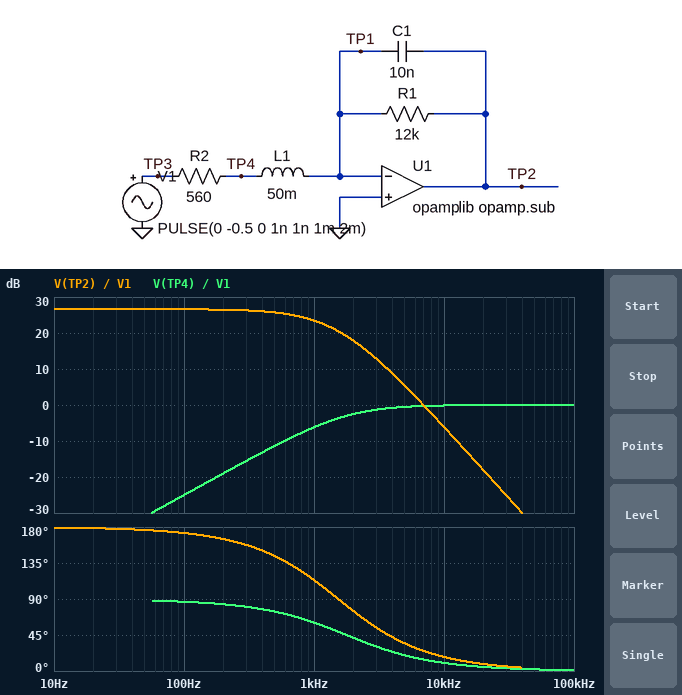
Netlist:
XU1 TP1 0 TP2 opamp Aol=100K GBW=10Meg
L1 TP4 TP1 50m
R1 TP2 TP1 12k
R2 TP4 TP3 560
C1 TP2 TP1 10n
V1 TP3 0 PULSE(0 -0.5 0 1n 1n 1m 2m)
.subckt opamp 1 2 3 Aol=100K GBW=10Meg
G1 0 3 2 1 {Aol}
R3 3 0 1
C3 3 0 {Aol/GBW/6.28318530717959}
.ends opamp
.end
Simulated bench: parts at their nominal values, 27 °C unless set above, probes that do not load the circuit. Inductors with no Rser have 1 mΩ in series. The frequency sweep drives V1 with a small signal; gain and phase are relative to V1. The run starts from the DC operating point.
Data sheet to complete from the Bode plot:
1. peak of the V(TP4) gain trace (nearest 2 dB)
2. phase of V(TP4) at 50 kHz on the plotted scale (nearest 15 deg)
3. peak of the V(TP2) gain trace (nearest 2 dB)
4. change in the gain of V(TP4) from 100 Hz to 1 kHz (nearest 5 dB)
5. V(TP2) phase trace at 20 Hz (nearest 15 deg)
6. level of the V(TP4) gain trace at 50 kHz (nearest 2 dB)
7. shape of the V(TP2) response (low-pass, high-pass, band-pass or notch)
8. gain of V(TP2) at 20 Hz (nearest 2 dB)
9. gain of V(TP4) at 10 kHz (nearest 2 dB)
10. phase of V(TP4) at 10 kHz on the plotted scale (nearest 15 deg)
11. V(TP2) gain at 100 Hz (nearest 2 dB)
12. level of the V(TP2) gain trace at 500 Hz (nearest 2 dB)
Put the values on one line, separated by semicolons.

0 dB; 0 deg; 26 dB; 20 dB; 180 deg; 0 dB; low-pass; 26 dB; 0 dB; 15 deg; 26 dB; 26 dB
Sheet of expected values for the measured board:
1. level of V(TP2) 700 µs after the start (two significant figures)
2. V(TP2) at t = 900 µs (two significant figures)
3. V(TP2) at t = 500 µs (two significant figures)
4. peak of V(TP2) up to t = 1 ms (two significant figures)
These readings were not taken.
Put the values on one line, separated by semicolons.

11 V; 11 V; 10 V; 11 V
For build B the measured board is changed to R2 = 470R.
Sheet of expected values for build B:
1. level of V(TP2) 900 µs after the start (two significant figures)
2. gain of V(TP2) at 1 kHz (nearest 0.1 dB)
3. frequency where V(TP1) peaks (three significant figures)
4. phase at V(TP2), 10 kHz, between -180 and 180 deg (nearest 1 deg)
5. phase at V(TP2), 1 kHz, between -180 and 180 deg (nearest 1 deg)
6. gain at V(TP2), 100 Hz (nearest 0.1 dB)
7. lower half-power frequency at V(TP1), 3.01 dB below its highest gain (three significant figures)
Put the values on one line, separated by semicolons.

13 V; 24.6 dB; 1.40 kHz; 16 deg; 109 deg; 28.1 dB; 572 Hz
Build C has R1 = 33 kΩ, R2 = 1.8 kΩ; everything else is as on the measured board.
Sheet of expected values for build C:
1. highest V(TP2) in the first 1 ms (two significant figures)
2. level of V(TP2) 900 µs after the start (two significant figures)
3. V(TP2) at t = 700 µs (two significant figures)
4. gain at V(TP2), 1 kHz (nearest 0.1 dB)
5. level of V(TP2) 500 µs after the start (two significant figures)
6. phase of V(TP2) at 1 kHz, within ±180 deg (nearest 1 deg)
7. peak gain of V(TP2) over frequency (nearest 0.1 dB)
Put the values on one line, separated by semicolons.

8.7 V; 8.5 V; 8.0 V; 17.9 dB; 7.0 V; 106 deg; 25.3 dB
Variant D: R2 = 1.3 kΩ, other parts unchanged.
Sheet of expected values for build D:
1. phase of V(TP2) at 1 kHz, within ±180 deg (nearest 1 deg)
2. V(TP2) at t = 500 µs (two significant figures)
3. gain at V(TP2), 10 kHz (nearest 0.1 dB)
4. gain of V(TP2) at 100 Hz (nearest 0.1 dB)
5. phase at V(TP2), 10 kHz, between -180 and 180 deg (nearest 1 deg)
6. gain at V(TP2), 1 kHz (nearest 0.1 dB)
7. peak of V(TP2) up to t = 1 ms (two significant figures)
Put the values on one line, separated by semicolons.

129 deg; 4.5 V; -6.7 dB; 19.3 dB; 30 deg; 17.1 dB; 4.6 V
